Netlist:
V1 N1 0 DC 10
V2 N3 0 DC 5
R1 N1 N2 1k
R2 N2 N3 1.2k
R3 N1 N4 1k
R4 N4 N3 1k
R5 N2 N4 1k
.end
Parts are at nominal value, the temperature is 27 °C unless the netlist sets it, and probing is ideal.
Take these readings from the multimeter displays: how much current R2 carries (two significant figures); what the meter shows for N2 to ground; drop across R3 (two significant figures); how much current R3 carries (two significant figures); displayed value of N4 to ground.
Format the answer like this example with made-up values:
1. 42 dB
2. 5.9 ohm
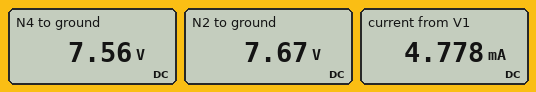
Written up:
1. 2.2 mA
2. 7.67 V
3. 2.4 V
4. 2.4 mA
5. 7.56 V
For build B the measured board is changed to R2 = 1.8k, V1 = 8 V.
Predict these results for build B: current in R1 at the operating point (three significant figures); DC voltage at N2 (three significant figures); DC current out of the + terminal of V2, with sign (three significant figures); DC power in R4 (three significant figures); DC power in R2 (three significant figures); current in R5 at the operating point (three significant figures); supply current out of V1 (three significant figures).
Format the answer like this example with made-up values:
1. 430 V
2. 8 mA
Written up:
1. 1.20 mA
2. 6.80 V
3. -2.60 mA
4. 2.56 mW
5. 1.80 mW
6. 200 µA
7. 2.60 mA
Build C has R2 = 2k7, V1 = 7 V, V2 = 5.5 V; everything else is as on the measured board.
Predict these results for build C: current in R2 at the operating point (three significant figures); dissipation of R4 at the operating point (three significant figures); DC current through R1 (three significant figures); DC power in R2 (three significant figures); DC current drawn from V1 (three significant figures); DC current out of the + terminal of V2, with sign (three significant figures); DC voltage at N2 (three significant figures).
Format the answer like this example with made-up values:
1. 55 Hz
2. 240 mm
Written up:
1. 364 µA
2. 684 µW
3. 518 µA
4. 357 µW
5. 1.19 mA
6. -1.19 mA
7. 6.48 V
